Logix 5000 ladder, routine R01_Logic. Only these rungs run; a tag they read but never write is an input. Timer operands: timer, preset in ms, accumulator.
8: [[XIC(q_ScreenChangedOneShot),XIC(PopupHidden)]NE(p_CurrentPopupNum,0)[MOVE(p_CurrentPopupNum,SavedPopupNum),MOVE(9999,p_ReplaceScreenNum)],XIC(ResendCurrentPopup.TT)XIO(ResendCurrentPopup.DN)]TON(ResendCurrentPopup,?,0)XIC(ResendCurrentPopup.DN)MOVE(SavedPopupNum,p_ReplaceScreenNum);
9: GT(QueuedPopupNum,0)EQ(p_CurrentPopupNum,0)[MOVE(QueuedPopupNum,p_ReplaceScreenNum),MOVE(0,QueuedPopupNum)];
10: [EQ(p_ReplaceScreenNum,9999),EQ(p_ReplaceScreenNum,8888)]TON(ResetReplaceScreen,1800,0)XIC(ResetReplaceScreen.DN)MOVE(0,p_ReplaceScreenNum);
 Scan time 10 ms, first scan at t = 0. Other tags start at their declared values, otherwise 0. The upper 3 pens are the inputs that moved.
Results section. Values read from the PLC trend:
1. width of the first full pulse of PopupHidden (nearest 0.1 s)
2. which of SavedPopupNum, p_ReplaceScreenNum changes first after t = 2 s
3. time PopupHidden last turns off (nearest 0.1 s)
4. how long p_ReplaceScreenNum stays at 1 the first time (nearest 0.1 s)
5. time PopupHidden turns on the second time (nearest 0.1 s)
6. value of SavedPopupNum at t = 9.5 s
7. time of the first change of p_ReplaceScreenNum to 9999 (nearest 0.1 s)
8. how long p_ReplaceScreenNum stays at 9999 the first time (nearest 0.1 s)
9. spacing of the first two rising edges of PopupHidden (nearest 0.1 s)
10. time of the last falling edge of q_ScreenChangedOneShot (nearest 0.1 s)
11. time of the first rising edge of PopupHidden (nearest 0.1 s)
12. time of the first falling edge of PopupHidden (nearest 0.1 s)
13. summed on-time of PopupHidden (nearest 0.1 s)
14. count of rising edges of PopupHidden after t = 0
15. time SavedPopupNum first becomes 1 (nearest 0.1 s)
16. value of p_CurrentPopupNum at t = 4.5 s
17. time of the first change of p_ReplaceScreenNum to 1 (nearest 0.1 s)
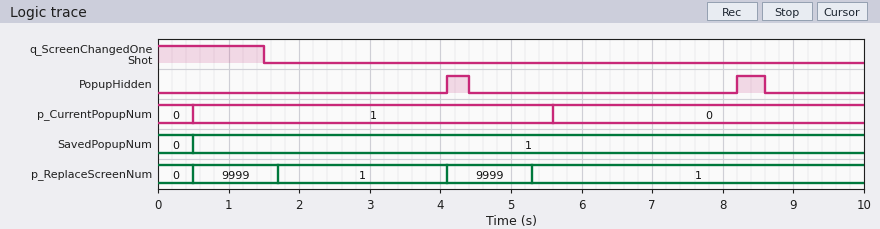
0.3 s
p_ReplaceScreenNum
8.6 s
2.4 s
8.2 s
1
0.5 s
1.2 s
4.1 s
1.5 s
4.1 s
4.4 s
0.7 s
2
0.5 s
1
1.7 s
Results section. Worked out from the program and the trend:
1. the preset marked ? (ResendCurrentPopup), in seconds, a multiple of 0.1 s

1.2 s
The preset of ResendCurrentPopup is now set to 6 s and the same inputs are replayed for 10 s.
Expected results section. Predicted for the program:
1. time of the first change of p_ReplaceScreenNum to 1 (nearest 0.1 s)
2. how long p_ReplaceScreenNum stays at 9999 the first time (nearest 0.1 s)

6.5 s
1.8 s
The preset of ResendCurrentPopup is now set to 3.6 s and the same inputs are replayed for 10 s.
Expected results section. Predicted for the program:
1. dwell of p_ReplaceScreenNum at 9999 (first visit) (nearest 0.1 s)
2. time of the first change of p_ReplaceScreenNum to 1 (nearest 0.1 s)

1.8 s
4.1 s
